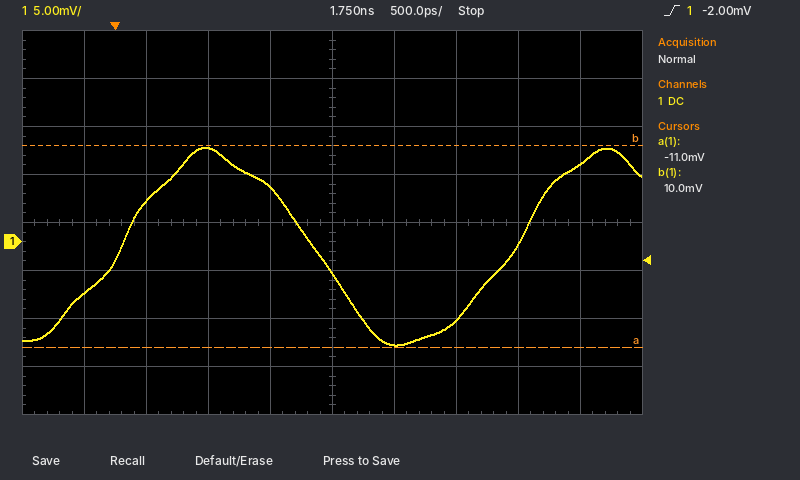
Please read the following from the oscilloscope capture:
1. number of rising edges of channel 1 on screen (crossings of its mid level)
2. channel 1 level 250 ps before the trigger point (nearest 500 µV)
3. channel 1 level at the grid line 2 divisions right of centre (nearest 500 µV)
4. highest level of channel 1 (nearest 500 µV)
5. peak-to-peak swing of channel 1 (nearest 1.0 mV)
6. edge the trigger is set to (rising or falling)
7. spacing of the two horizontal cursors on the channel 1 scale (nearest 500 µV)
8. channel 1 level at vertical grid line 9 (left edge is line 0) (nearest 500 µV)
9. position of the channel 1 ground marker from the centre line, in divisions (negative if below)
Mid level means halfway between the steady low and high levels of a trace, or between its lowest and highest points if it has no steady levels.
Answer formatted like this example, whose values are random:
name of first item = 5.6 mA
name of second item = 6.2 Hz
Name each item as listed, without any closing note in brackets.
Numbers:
number of rising edges of channel 1 on screen = 2
channel 1 level 250 ps before the trigger point = -5.5 mV
channel 1 level at the grid line 2 divisions right of centre = -8.0 mV
highest level of channel 1 = 10.0 mV
peak-to-peak swing of channel 1 = 21.0 mV
edge the trigger is set to = rising
spacing of the two horizontal cursors on the channel 1 scale = 21.0 mV
channel 1 level at vertical grid line 9 (left edge is line 0) = 8.0 mV
position of the channel 1 ground marker from the centre line, in divisions = -0.4 div
